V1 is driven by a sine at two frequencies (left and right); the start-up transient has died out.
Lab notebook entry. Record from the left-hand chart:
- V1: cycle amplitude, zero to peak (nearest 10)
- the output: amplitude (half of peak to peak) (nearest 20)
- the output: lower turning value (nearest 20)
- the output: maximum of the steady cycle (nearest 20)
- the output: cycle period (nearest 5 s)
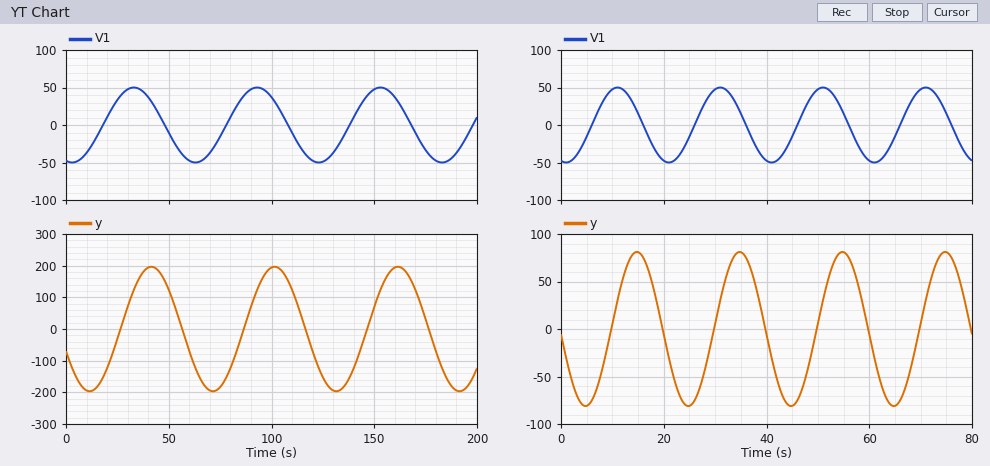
50
200
-200
200
60 s
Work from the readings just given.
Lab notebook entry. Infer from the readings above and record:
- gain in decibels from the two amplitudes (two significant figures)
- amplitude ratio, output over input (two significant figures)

12 dB
4.0
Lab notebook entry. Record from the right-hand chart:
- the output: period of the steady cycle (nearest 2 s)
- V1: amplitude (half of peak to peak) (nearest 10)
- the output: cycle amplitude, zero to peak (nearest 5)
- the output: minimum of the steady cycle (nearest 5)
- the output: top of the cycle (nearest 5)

20 s
50
80
-80
80
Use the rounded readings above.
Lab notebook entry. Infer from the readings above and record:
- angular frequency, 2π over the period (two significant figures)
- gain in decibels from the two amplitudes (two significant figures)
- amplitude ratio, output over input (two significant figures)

0.31 rad/s
4.1 dB
1.6
